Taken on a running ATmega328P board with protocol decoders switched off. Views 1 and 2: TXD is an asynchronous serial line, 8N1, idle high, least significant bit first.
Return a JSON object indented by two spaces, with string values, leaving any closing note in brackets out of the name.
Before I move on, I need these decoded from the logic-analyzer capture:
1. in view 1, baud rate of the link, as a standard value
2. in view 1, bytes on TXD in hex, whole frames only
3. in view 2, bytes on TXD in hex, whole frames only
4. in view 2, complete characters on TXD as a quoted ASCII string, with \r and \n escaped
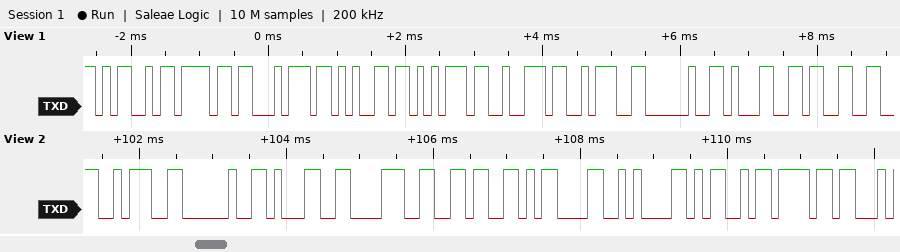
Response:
{
  "in view 1, baud rate of the link, as a standard value": "9600 baud",
  "in view 1, bytes on TXD in hex, whole frames only": "4D 6F 74 65 75 72 3A 20 31 33",
  "in view 2, bytes on TXD in hex, whole frames only": "0x3A 0x20 0x31 0x38 0x36 0x0D 0x0A 0x4D 0x6F",
  "in view 2, complete characters on TXD as a quoted ASCII string, with \\r and \\n escaped": "\": 186\\r\\nMo\""
}
